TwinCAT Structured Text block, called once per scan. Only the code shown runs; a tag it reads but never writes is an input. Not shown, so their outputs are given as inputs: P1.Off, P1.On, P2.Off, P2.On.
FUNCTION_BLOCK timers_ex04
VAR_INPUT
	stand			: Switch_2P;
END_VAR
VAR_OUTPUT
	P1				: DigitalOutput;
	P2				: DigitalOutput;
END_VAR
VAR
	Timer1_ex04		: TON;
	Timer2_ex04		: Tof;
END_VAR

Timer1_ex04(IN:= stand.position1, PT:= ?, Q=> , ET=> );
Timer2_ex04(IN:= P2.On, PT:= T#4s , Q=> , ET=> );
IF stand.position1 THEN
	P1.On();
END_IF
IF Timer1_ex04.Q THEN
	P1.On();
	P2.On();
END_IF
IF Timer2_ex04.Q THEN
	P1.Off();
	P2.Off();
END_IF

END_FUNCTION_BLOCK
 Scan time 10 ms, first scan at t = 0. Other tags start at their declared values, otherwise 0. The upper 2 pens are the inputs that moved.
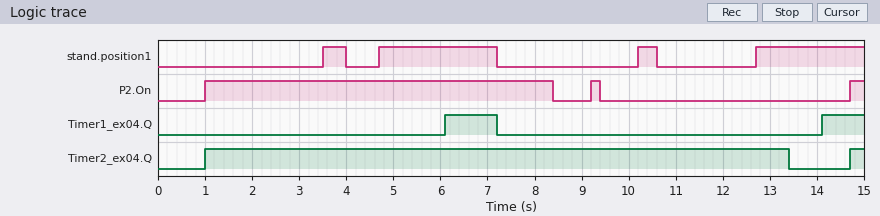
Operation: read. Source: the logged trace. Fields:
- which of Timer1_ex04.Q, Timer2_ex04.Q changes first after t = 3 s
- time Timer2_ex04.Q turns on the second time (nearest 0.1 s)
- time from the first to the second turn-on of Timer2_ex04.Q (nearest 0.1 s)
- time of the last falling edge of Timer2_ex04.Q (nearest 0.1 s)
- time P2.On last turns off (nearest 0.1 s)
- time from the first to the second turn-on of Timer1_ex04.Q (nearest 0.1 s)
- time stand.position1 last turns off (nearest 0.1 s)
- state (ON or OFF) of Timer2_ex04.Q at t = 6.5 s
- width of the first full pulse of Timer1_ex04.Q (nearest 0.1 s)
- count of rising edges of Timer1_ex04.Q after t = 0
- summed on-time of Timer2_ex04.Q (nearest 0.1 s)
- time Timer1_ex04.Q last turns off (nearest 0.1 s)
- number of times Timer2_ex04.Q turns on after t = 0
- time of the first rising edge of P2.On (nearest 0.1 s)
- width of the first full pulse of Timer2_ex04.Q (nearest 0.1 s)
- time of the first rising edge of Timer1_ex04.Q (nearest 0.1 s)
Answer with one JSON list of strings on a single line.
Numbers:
["Timer1_ex04.Q", "14.7 s", "13.7 s", "13.4 s", "9.4 s", "8.0 s", "10.6 s", "ON", "1.1 s", "2", "12.7 s", "7.2 s", "2", "1.0 s", "12.4 s", "6.1 s"]
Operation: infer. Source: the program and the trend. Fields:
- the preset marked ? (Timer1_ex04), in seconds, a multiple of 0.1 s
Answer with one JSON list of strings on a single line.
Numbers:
["1.4 s"]
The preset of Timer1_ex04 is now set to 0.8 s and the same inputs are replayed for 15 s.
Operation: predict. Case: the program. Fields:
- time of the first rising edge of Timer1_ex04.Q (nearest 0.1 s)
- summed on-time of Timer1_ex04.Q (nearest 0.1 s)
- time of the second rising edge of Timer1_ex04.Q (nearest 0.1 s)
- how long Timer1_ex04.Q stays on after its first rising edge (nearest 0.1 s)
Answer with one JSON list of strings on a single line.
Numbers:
["5.5 s", "3.2 s", "13.5 s", "1.7 s"]
